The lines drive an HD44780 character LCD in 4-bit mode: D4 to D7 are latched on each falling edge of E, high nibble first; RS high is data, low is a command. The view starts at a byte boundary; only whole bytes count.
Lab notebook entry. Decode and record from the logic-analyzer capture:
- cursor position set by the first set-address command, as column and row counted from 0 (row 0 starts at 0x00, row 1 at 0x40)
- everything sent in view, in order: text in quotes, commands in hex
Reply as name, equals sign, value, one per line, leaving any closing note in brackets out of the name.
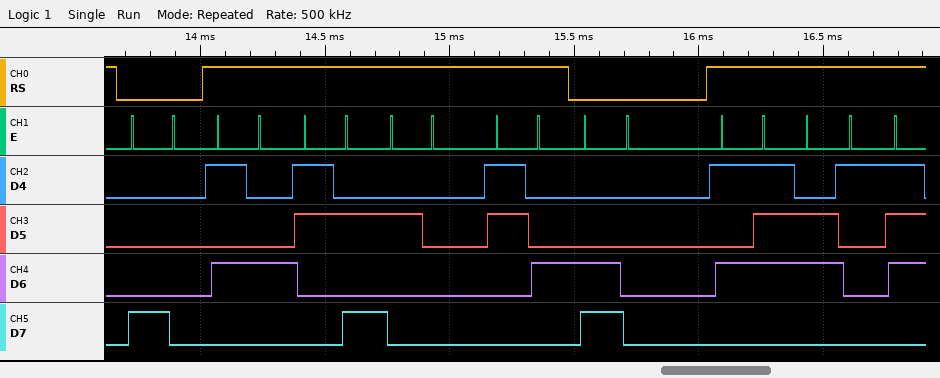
cursor position set by the first set-address command, as column and row counted from 0 = column 0, row 0
everything sent in view, in order: text in quotes, commands in hex = 0x80 "T: 4" 0xC0 "Wa"
